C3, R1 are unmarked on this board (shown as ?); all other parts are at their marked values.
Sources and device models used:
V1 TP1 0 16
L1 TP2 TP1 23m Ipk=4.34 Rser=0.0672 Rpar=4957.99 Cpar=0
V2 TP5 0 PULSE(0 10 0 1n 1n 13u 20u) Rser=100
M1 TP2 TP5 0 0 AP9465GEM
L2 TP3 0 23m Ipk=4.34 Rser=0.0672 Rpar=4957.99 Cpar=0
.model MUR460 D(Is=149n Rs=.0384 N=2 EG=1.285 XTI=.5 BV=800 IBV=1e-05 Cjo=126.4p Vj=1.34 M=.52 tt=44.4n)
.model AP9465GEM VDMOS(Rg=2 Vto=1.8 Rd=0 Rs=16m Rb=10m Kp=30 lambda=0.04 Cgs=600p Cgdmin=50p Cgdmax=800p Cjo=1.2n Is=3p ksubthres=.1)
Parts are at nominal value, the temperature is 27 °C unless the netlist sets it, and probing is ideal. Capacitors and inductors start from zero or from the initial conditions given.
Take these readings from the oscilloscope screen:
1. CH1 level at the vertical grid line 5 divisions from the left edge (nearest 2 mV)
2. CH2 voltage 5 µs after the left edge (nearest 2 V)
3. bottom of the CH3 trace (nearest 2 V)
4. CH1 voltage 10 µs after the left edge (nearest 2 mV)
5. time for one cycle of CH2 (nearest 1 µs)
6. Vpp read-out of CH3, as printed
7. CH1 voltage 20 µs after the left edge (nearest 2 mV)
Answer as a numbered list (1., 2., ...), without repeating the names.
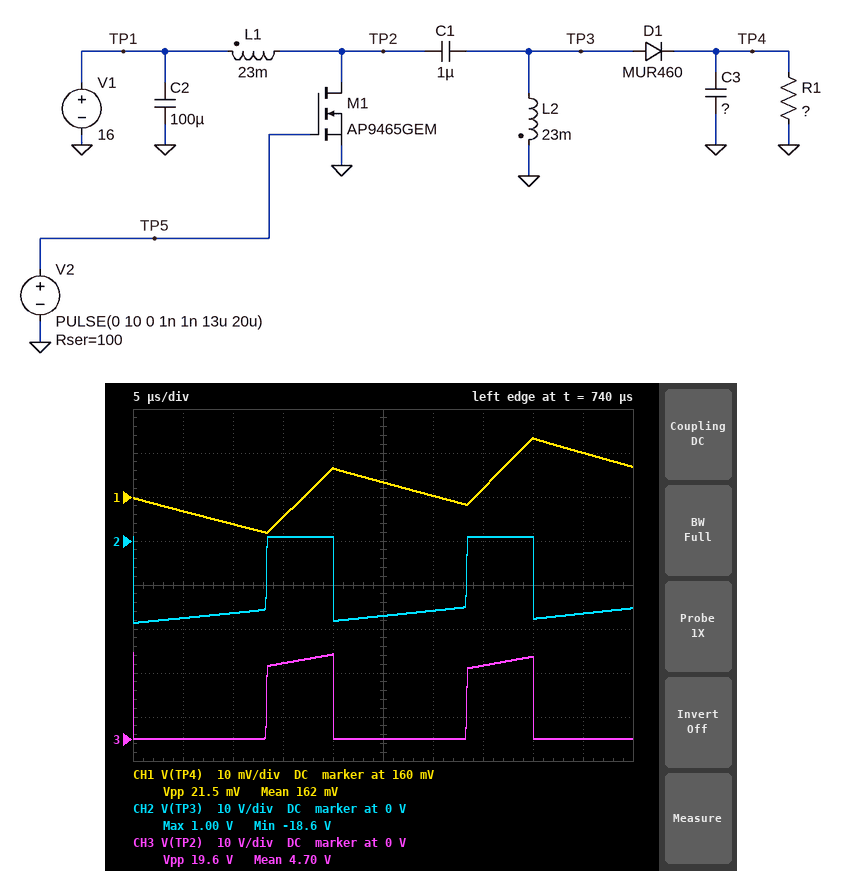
1. 164 mV
2. -18 V
3. 0 V
4. 154 mV
5. 20 µs
6. 19.6 V
7. 166 mV
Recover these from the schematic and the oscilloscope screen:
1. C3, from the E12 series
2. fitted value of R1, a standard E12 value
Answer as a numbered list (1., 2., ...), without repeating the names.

1. 220 µF
2. 1.2 Ω
